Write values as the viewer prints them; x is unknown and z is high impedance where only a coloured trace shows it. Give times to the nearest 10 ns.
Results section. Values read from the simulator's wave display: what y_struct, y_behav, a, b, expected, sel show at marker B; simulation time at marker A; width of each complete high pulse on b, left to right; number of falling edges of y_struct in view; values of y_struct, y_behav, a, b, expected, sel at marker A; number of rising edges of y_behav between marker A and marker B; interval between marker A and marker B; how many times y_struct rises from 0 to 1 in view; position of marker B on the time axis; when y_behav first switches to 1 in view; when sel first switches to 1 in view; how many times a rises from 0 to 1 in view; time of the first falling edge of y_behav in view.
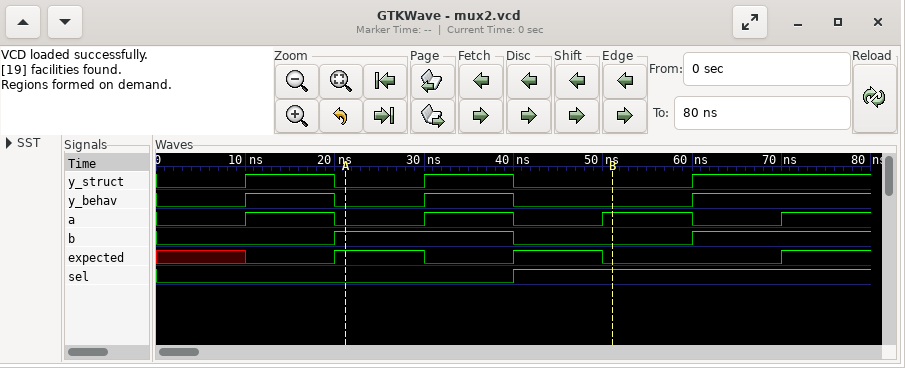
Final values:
y_struct=0, y_behav=0, a=1, b=0, expected=0, sel=1
20 ns
20 ns
2
y_struct=0, y_behav=0, a=0, b=1, expected=1, sel=0
1
30 ns
3
50 ns
10 ns
40 ns
4
20 ns
